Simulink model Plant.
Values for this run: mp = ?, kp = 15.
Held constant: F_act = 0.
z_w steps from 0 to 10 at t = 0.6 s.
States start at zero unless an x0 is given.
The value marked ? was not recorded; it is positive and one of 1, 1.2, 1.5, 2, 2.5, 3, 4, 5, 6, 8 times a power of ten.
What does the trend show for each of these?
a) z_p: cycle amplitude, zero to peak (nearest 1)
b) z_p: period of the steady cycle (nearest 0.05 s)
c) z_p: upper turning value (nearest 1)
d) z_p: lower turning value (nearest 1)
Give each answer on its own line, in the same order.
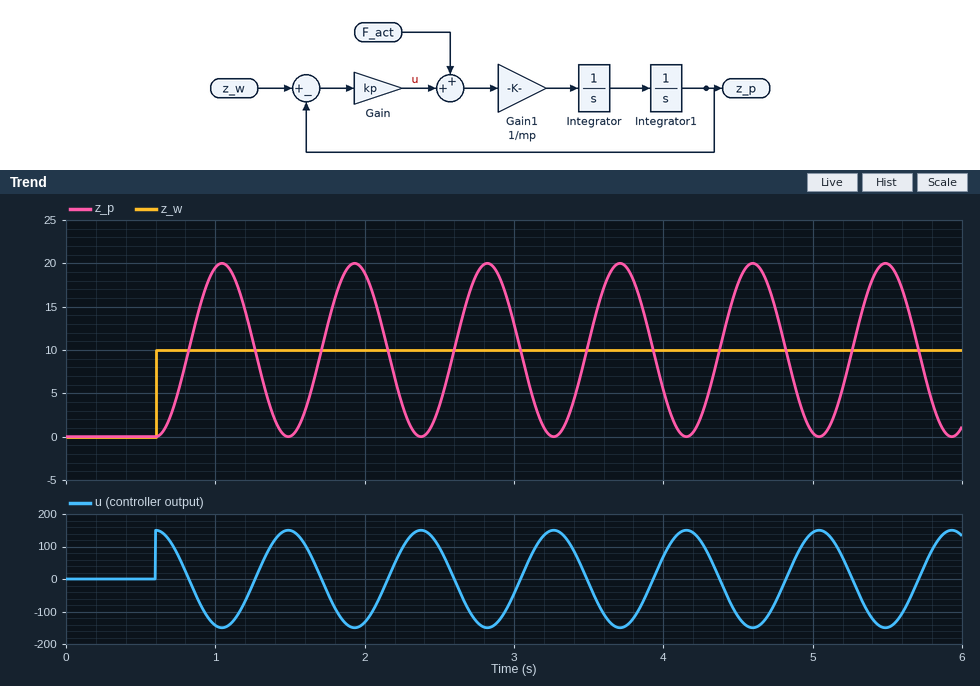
10
0.90 s
20
0
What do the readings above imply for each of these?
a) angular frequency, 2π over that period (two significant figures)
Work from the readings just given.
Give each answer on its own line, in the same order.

7.0 rad/s
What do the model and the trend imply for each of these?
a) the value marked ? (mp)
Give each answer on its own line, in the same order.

0.3
